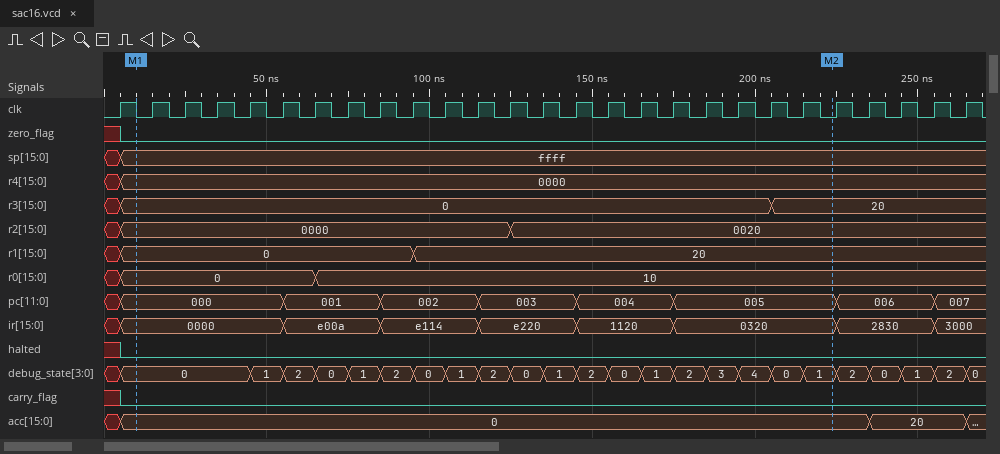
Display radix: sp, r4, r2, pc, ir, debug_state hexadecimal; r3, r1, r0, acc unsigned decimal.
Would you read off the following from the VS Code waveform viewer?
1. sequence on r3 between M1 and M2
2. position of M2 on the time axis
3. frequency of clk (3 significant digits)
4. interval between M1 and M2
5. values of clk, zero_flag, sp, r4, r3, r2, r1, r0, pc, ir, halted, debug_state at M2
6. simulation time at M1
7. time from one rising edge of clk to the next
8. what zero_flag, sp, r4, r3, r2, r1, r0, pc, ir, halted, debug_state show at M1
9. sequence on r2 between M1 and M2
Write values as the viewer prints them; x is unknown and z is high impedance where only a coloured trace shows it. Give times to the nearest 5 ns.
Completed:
0, 20
225 ns
100 MHz
215 ns
clk=0, zero_flag=0, sp=ffff, r4=0000, r3=20, r2=0020, r1=20, r0=10, pc=005, ir=0320, halted=0, debug_state=1
10 ns
10 ns
zero_flag=0, sp=ffff, r4=0000, r3=0, r2=0000, r1=0, r0=0, pc=000, ir=0000, halted=0, debug_state=0
0000, 0020
